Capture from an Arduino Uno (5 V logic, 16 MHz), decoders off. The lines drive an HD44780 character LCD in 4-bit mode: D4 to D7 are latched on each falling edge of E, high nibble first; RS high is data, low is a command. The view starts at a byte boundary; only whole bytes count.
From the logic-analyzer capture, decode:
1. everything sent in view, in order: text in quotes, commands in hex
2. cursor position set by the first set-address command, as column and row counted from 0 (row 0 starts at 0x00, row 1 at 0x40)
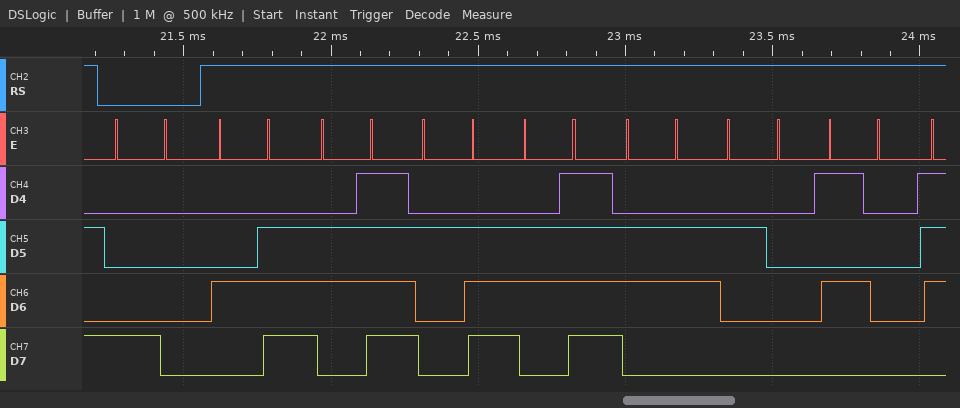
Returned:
0x80 "No.of P"
column 0, row 0
